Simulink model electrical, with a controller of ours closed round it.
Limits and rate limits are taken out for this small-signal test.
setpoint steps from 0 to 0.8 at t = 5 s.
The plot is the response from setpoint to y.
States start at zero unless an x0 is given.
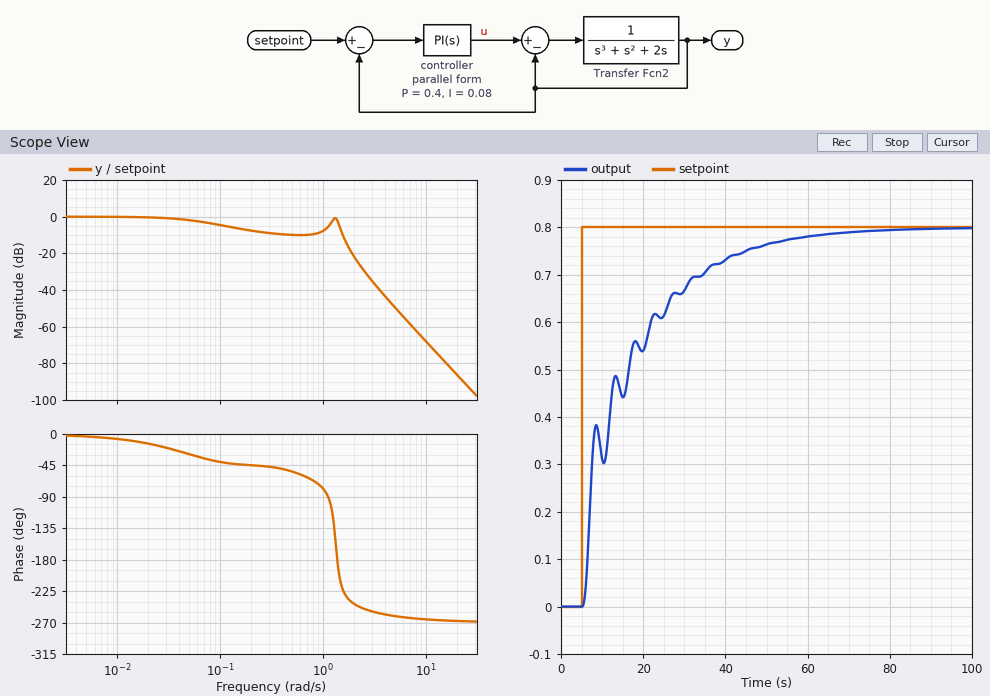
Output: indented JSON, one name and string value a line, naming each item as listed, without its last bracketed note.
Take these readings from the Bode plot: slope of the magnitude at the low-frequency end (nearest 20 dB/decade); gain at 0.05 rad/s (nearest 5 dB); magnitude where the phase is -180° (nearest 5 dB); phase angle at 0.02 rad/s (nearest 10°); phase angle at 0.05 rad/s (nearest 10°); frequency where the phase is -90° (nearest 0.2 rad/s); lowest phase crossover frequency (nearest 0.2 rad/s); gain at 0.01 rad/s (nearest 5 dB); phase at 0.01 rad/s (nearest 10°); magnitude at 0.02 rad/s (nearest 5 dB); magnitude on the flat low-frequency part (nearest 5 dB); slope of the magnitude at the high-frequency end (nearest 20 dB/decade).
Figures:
{
  "slope of the magnitude at the low-frequency end": "0 dB/decade",
  "gain at 0.05 rad/s": "0 dB",
  "magnitude where the phase is -180°": "0 dB",
  "phase angle at 0.02 rad/s": "-10°",
  "phase angle at 0.05 rad/s": "-30°",
  "frequency where the phase is -90°": "1.2 rad/s",
  "lowest phase crossover frequency": "1.4 rad/s",
  "gain at 0.01 rad/s": "0 dB",
  "phase at 0.01 rad/s": "-10°",
  "magnitude at 0.02 rad/s": "0 dB",
  "magnitude on the flat low-frequency part": "0 dB",
  "slope of the magnitude at the high-frequency end": "-60 dB/decade"
}
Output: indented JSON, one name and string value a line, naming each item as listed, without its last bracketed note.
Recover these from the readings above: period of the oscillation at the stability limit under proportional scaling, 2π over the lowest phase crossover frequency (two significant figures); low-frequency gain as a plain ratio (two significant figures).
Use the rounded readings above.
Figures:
{
  "period of the oscillation at the stability limit under proportional scaling, 2π over the lowest phase crossover frequency": "4.5 s",
  "low-frequency gain as a plain ratio": "1.0"
}
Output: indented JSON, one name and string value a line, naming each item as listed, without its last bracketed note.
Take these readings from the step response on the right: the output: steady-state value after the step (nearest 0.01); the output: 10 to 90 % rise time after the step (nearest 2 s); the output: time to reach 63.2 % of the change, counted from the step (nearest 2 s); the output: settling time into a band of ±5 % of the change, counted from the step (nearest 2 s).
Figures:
{
  "the output: steady-state value after the step": "0.80",
  "the output: 10 to 90 % rise time after the step": "30 s",
  "the output: time to reach 63.2 % of the change, counted from the step": "12 s",
  "the output: settling time into a band of ±5 % of the change, counted from the step": "44 s"
}
